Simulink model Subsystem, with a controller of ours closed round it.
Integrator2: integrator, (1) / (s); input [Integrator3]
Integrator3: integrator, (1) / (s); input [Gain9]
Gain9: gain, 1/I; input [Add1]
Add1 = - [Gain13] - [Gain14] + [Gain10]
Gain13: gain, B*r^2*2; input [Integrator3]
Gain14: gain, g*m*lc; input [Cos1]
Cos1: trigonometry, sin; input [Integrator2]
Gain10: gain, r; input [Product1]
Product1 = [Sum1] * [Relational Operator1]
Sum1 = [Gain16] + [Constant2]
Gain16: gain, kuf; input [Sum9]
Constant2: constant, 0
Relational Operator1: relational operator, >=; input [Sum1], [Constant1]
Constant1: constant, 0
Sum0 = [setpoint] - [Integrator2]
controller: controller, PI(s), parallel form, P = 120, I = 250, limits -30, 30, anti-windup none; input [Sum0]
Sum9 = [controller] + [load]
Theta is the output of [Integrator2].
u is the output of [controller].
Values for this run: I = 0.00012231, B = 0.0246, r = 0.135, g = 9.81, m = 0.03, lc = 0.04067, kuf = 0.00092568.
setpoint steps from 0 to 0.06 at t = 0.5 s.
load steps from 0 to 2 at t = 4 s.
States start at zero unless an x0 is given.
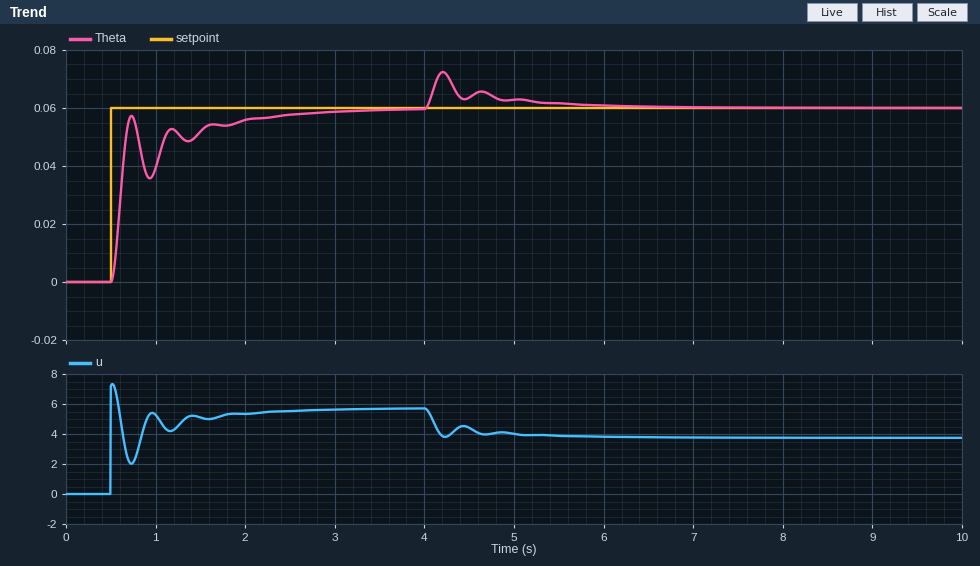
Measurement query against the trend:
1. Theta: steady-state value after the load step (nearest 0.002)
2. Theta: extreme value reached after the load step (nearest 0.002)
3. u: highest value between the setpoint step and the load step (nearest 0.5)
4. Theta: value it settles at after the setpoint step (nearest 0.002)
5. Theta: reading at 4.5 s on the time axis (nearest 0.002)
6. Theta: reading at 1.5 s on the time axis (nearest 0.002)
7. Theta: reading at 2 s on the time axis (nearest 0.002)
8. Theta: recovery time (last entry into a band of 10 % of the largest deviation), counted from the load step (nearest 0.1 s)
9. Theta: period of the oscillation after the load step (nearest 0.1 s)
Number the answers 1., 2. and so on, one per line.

1. 0.060
2. 0.072
3. 7.5
4. 0.060
5. 0.064
6. 0.052
7. 0.056
8. 1.7 s
9. 0.4 s
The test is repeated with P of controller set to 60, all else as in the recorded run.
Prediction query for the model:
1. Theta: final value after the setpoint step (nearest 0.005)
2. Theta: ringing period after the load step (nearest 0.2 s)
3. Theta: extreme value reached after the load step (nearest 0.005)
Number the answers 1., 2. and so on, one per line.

1. 0.060
2. 0.6 s
3. 0.075
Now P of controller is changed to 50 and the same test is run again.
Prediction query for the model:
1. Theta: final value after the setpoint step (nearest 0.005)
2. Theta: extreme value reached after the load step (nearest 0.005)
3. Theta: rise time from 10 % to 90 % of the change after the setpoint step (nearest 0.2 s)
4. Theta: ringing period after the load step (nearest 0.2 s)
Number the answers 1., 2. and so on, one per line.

1. 0.060
2. 0.075
3. 0.8 s
4. 0.6 s
